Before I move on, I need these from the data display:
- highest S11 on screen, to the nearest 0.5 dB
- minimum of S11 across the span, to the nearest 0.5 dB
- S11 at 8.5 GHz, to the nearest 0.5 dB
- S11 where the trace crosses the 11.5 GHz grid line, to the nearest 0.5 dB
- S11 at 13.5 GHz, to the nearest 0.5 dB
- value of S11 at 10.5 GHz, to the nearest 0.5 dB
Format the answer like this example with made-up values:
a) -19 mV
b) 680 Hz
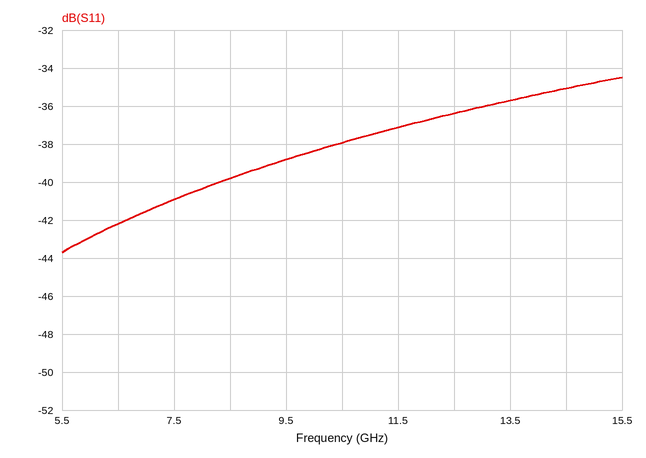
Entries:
a) -34.5 dB
b) -43.5 dB
c) -40.0 dB
d) -37.0 dB
e) -35.5 dB
f) -38.0 dB
